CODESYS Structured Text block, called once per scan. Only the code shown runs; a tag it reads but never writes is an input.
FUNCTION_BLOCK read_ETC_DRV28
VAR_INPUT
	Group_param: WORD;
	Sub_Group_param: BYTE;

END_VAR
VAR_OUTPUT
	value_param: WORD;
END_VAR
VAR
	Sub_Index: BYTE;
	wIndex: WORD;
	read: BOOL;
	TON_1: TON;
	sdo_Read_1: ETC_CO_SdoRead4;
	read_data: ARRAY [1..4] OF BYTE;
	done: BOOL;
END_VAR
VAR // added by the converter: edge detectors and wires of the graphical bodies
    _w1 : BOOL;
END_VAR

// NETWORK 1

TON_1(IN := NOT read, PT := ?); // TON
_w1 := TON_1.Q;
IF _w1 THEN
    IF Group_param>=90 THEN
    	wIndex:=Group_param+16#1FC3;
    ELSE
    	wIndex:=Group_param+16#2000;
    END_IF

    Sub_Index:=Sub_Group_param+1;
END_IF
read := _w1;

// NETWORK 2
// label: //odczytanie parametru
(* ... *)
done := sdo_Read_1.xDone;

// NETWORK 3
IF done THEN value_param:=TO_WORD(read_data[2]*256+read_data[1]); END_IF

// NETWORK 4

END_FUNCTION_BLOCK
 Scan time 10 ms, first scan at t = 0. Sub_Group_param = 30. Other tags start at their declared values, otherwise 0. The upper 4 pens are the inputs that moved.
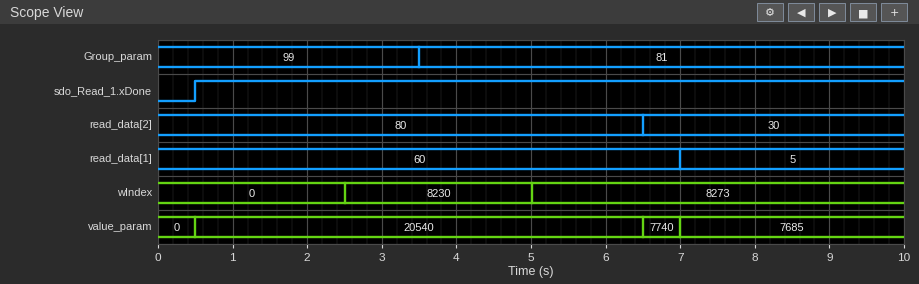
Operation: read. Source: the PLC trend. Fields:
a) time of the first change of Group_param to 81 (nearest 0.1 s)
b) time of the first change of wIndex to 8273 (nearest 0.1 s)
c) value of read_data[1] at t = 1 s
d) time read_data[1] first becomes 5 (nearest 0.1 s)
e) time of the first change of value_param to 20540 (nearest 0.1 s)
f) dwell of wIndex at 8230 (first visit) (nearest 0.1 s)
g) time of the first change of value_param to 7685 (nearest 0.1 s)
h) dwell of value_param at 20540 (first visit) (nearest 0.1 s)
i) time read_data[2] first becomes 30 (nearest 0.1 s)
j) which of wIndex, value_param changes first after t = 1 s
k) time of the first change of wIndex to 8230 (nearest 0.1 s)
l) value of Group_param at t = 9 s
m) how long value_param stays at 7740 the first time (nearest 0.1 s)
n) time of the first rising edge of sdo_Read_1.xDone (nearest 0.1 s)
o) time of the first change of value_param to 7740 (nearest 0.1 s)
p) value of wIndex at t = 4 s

3.5 s
5.0 s
60
7.0 s
0.5 s
2.5 s
7.0 s
6.0 s
6.5 s
wIndex
2.5 s
81
0.5 s
0.5 s
6.5 s
8230
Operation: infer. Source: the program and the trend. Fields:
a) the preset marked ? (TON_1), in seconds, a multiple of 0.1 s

2.5 s
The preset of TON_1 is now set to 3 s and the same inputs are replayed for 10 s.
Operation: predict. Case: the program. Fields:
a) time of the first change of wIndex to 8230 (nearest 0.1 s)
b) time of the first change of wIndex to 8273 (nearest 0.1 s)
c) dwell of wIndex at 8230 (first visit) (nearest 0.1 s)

3.0 s
6.0 s
3.0 s
